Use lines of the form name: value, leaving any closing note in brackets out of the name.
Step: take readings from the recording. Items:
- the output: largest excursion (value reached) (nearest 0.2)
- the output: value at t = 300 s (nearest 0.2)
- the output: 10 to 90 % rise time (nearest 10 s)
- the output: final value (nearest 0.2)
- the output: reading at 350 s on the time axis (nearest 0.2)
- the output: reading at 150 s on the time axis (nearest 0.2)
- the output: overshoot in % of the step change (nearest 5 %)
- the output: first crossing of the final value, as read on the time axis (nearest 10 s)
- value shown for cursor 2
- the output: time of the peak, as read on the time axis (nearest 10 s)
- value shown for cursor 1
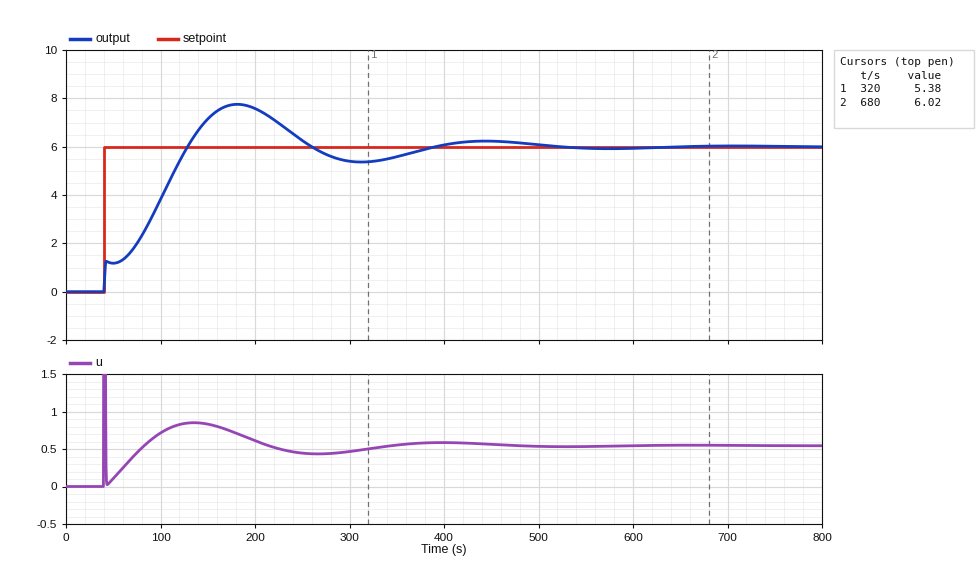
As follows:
the output: largest excursion (value reached): 7.8
the output: value at t = 300 s: 5.4
the output: 10 to 90 % rise time: 80 s
the output: final value: 6.0
the output: reading at 350 s on the time axis: 5.6
the output: reading at 150 s on the time axis: 7.2
the output: overshoot in % of the step change: 30 %
the output: first crossing of the final value, as read on the time axis: 130 s
value shown for cursor 2: 6.02
the output: time of the peak, as read on the time axis: 180 s
value shown for cursor 1: 5.38
